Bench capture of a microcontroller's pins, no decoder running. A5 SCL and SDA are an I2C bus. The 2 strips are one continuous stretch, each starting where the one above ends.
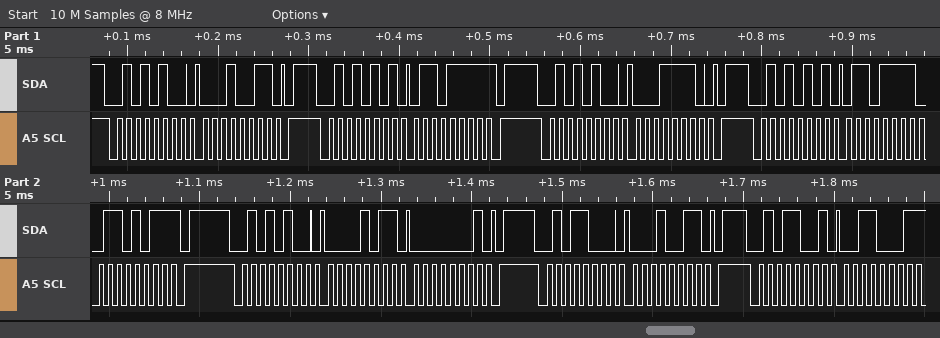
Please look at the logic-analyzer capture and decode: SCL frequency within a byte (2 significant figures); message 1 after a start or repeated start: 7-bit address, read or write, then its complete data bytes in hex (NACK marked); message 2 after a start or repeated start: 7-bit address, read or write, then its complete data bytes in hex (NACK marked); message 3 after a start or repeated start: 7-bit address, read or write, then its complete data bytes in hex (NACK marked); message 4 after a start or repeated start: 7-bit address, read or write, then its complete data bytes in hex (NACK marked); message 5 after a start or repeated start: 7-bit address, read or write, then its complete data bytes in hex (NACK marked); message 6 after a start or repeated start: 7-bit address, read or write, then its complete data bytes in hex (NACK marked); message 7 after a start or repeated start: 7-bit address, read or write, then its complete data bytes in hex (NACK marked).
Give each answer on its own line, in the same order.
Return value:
100 kHz
0x2A write: 13
0x2A read: 6F NACK
0x2A write: 1E
0x2A read: 6F 6B NACK
0x2A write: 0B 01
0x2C write: 13
0x2C read: 31 NACK
